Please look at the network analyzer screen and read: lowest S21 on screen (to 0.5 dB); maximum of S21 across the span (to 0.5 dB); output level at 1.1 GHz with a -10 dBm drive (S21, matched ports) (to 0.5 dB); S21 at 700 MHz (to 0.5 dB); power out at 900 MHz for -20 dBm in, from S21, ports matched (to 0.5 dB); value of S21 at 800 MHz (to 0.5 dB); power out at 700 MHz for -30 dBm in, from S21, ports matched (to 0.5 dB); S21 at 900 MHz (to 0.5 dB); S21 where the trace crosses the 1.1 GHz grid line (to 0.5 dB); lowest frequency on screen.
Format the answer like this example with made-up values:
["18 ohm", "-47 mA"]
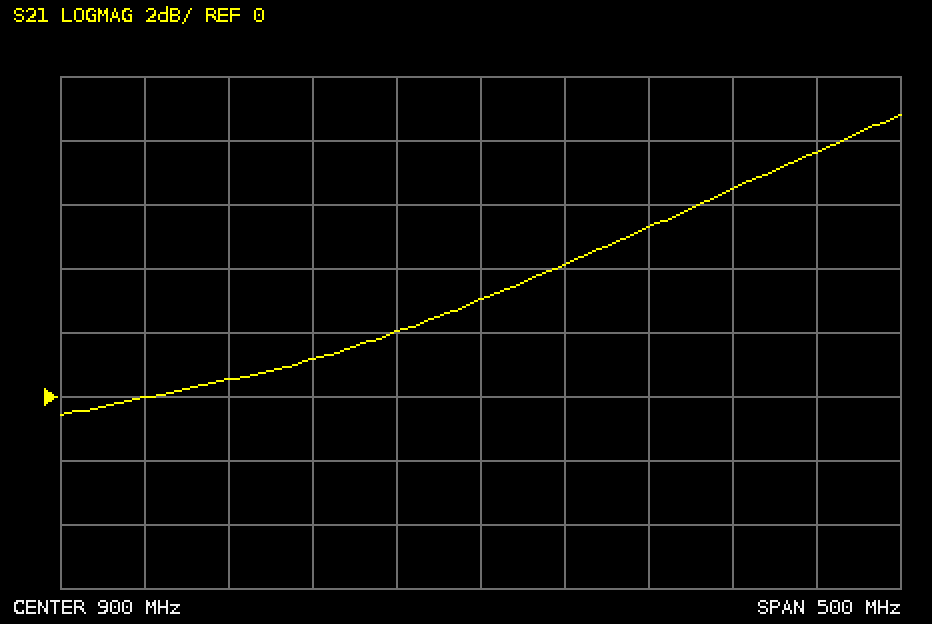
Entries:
["-0.5 dB", "9.0 dB", "-2.5 dBm", "0.0 dB", "-17.0 dBm", "1.0 dB", "-30.0 dBm", "3.0 dB", "7.5 dB", "650 MHz"]
